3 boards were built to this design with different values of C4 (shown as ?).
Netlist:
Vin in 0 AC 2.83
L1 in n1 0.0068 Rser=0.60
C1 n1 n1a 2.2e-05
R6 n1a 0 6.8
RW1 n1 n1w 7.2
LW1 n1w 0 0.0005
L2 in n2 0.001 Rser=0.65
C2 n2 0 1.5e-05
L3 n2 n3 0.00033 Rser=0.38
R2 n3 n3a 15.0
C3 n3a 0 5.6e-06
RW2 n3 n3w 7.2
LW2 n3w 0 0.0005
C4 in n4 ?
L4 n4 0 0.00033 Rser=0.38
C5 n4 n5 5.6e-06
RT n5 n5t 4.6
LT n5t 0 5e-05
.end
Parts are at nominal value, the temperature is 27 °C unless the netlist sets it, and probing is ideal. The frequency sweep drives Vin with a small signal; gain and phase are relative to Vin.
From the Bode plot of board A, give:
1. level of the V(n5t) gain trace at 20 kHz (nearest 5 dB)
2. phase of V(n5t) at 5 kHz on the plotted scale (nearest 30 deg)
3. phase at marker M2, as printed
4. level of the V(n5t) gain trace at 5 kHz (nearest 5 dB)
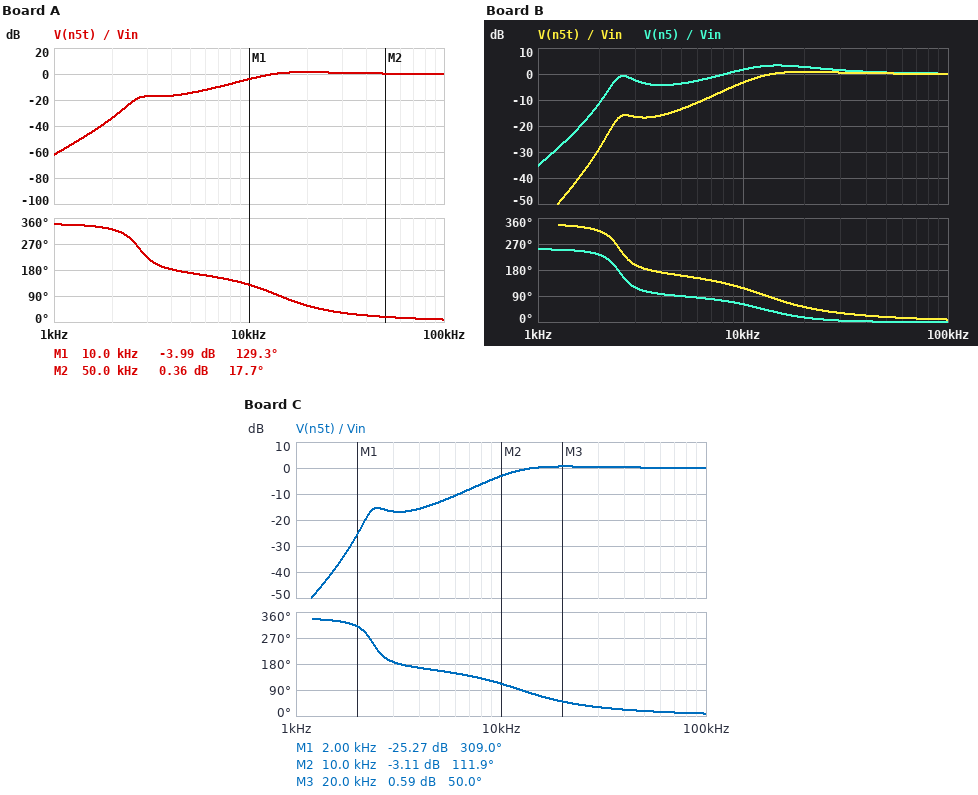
0 dB
180 deg
17.7 deg
-15 dB
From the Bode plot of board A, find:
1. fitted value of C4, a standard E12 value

4.7 µF
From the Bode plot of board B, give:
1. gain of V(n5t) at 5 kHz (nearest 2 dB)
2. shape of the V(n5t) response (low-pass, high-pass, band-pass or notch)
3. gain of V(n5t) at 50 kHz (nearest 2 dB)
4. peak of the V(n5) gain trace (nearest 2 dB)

-14 dB
high-pass
0 dB
4 dB
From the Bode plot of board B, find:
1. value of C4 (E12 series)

6.8 µF
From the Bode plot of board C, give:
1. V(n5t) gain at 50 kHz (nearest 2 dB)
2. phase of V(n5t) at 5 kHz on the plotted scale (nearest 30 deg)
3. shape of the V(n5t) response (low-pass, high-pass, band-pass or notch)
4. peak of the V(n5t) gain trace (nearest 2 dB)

0 dB
150 deg
high-pass
0 dB
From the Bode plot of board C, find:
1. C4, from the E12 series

8.2 µF
